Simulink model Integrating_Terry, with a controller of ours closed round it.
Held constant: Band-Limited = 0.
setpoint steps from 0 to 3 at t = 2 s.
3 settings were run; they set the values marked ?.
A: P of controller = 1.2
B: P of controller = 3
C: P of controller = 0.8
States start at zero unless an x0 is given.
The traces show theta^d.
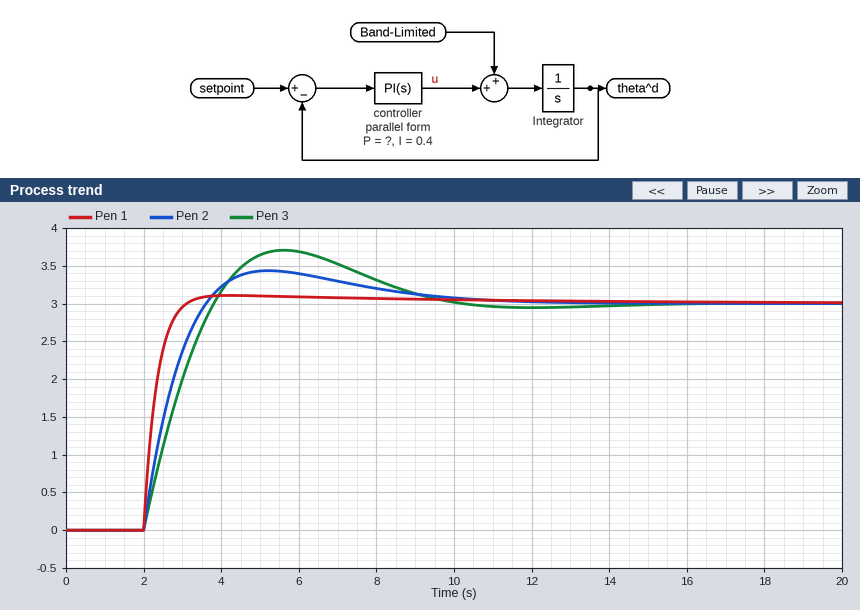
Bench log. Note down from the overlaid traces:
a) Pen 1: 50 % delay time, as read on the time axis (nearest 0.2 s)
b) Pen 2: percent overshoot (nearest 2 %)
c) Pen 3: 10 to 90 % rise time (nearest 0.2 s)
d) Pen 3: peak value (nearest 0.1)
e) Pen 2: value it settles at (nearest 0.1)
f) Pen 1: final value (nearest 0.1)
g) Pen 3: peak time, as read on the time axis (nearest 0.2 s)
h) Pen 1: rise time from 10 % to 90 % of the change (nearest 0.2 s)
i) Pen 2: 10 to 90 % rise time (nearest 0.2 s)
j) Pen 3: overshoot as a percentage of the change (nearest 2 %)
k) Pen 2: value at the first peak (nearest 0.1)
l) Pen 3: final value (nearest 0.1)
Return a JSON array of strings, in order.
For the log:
["2.2 s", "14 %", "1.4 s", "3.7", "3.0", "3.0", "5.6 s", "0.6 s", "1.2 s", "24 %", "3.4", "3.0"]
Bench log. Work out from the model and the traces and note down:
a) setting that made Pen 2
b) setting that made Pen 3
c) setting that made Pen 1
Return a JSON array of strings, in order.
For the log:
["A", "C", "B"]
